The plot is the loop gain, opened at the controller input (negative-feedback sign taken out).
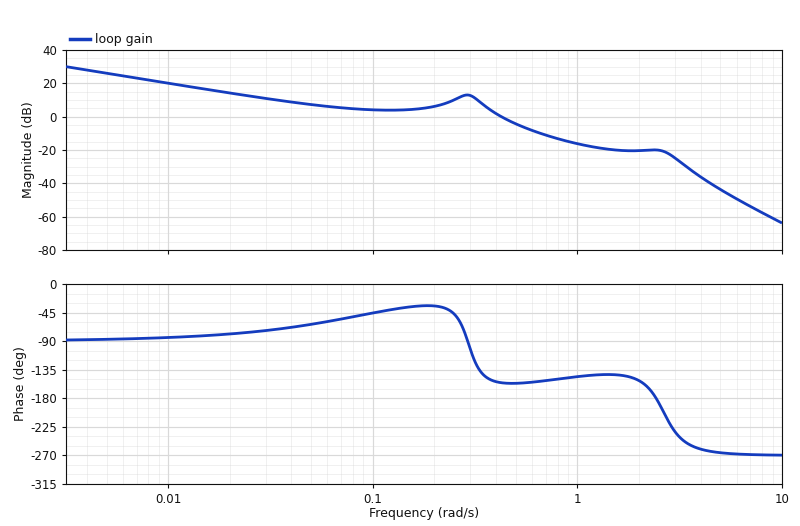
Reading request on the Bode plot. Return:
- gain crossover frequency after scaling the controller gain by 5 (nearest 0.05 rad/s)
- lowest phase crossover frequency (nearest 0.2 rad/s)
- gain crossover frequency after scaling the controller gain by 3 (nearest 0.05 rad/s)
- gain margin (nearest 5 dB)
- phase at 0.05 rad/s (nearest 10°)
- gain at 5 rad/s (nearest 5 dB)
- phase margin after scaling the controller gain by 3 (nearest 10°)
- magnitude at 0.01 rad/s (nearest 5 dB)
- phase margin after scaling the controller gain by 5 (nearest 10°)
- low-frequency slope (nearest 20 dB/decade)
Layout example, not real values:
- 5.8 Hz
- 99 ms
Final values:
- 0.85 rad/s
- 2.4 rad/s
- 0.65 rad/s
- 20 dB
- -60°
- -45 dB
- 30°
- 20 dB
- 30°
- -20 dB/decade
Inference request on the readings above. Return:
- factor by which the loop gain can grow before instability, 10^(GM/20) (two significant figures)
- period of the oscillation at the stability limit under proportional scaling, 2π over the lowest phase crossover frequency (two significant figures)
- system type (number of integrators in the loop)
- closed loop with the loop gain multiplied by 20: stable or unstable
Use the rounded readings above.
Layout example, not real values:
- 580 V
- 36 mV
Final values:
- 10
- 2.6 s
- 1
- unstable
